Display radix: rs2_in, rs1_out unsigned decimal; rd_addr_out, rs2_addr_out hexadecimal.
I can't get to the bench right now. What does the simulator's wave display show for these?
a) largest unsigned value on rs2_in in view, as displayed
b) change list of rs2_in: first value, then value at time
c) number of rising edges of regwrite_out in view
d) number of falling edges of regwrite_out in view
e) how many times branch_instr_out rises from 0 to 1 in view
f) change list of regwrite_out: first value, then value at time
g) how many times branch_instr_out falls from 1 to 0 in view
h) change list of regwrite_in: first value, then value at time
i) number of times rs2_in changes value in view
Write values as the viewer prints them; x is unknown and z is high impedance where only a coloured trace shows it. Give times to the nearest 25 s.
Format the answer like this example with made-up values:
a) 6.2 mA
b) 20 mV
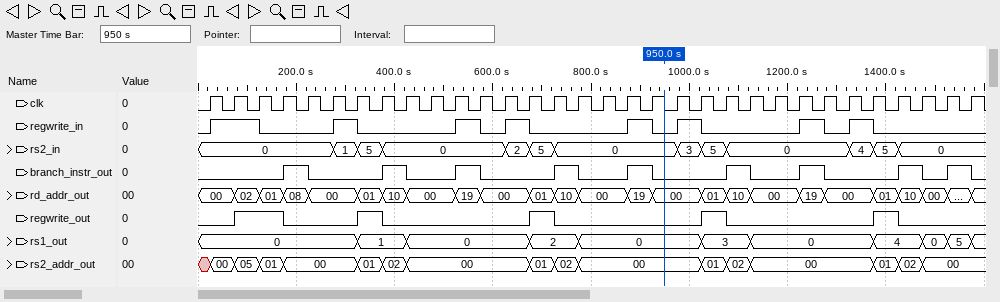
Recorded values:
a) 5
b) 0, 1 at 275 s, 5 at 325 s, 0 at 375 s, 2 at 625 s, 5 at 675 s, 0 at 725 s, 3 at 975 s, 5 at 1025 s, 0 at 1075 s, 4 at 1325 s, 5 at 1375 s, 0 at 1425 s
c) 5
d) 5
e) 9
f) 0, 1 at 75 s, 0 at 175 s, 1 at 325 s, 0 at 375 s, 1 at 675 s, 0 at 725 s, 1 at 1025 s, 0 at 1075 s, 1 at 1375 s, 0 at 1425 s
g) 9
h) 0, 1 at 25 s, 0 at 125 s, 1 at 275 s, 0 at 325 s, 1 at 525 s, 0 at 575 s, 1 at 625 s, 0 at 675 s, 1 at 875 s, 0 at 925 s, 1 at 975 s, 0 at 1025 s, 1 at 1225 s, 0 at 1275 s, 1 at 1325 s, 0 at 1375 s
i) 12
